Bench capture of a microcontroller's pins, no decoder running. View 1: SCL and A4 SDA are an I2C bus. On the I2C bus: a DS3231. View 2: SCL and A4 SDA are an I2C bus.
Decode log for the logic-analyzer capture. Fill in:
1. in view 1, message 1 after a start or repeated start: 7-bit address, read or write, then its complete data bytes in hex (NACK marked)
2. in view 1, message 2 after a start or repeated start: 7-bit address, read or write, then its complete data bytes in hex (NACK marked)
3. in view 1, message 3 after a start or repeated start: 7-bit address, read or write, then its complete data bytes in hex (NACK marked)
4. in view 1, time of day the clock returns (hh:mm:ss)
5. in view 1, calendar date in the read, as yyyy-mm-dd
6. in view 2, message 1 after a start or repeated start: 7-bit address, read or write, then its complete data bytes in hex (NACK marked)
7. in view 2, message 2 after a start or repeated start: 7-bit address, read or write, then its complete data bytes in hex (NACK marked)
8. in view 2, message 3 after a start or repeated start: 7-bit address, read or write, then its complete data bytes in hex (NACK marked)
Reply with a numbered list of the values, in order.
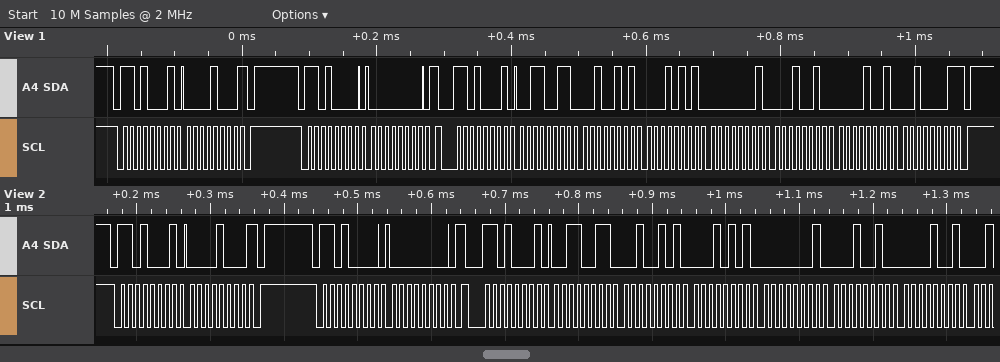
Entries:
1. 0x68 read: 08 NACK
2. 0x68 write: 00
3. 0x68 read: 33 25 15 01 12 09 21 NACK
4. 15:25:33
5. 2021-09-12
6. 0x68 read: 08 NACK
7. 0x68 write: 00
8. 0x68 read: 33 25 15 01 12 09
